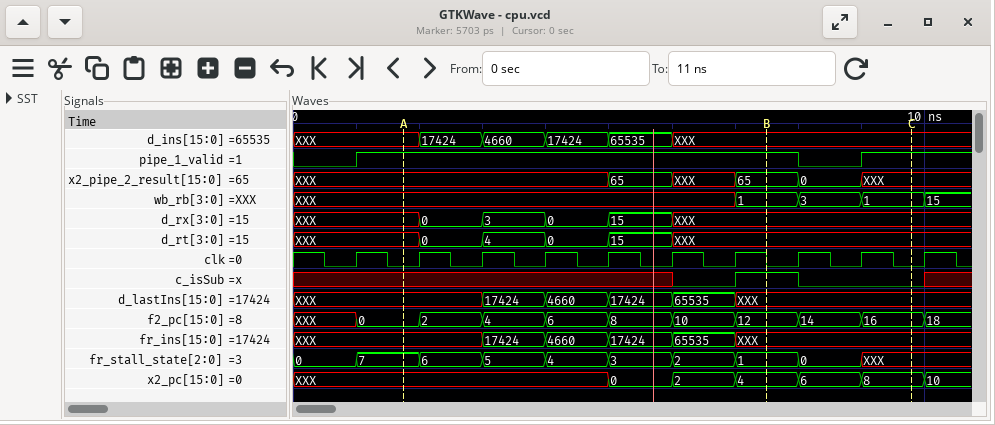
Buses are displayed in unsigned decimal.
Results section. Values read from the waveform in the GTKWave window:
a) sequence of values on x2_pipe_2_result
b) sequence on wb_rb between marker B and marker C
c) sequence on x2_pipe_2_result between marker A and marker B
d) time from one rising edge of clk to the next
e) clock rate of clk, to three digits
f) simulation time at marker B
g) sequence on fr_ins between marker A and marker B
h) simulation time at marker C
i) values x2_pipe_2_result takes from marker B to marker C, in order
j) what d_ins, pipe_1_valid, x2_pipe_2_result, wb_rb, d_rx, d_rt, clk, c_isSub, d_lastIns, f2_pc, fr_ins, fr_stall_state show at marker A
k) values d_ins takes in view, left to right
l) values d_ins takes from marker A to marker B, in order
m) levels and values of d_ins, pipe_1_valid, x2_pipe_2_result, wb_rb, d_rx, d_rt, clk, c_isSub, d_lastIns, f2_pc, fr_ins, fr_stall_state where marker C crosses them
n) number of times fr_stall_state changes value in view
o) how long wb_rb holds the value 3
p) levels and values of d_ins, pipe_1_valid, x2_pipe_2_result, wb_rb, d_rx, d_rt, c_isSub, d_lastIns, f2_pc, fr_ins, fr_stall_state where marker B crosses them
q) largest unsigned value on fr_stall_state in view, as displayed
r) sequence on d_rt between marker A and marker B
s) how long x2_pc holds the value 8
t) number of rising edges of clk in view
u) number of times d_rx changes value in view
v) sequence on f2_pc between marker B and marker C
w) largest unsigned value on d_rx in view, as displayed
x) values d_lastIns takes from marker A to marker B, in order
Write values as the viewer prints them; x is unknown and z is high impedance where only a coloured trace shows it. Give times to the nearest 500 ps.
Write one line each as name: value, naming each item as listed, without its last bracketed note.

sequence of values on x2_pipe_2_result: XXX, 65, XXX, 65, 0, XXX
sequence on wb_rb between marker B and marker C: 1, 3, 1
sequence on x2_pipe_2_result between marker A and marker B: XXX, 65, XXX, 65
time from one rising edge of clk to the next: 1000 ps
clock rate of clk, to three digits: 1.00 GHz
simulation time at marker B: 7500 ps
sequence on fr_ins between marker A and marker B: XXX, 17424, 4660, 17424, 65535, XXX
simulation time at marker C: 10000 ps
values x2_pipe_2_result takes from marker B to marker C, in order: 65, 0, XXX
what d_ins, pipe_1_valid, x2_pipe_2_result, wb_rb, d_rx, d_rt, clk, c_isSub, d_lastIns, f2_pc, fr_ins, fr_stall_state show at marker A: d_ins=XXX, pipe_1_valid=1, x2_pipe_2_result=XXX, wb_rb=XXX, d_rx=XXX, d_rt=XXX, clk=0, c_isSub=x, d_lastIns=XXX, f2_pc=0, fr_ins=XXX, fr_stall_state=7
values d_ins takes in view, left to right: XXX, 17424, 4660, 17424, 65535, XXX
values d_ins takes from marker A to marker B, in order: XXX, 17424, 4660, 17424, 65535, XXX
levels and values of d_ins, pipe_1_valid, x2_pipe_2_result, wb_rb, d_rx, d_rt, clk, c_isSub, d_lastIns, f2_pc, fr_ins, fr_stall_state where marker C crosses them: d_ins=XXX, pipe_1_valid=1, x2_pipe_2_result=XXX, wb_rb=1, d_rx=XXX, d_rt=XXX, clk=0, c_isSub=0, d_lastIns=XXX, f2_pc=16, fr_ins=XXX, fr_stall_state=XXX
number of times fr_stall_state changes value in view: 9
how long wb_rb holds the value 3: 1000 ps
levels and values of d_ins, pipe_1_valid, x2_pipe_2_result, wb_rb, d_rx, d_rt, c_isSub, d_lastIns, f2_pc, fr_ins, fr_stall_state where marker B crosses them: d_ins=XXX, pipe_1_valid=1, x2_pipe_2_result=65, wb_rb=1, d_rx=XXX, d_rt=XXX, c_isSub=1, d_lastIns=XXX, f2_pc=12, fr_ins=XXX, fr_stall_state=1
largest unsigned value on fr_stall_state in view, as displayed: 7
sequence on d_rt between marker A and marker B: XXX, 0, 4, 0, 15, XXX
how long x2_pc holds the value 8: 1000 ps
number of rising edges of clk in view: 10
number of times d_rx changes value in view: 5
sequence on f2_pc between marker B and marker C: 12, 14, 16
largest unsigned value on d_rx in view, as displayed: 15
values d_lastIns takes from marker A to marker B, in order: XXX, 17424, 4660, 17424, 65535, XXX
